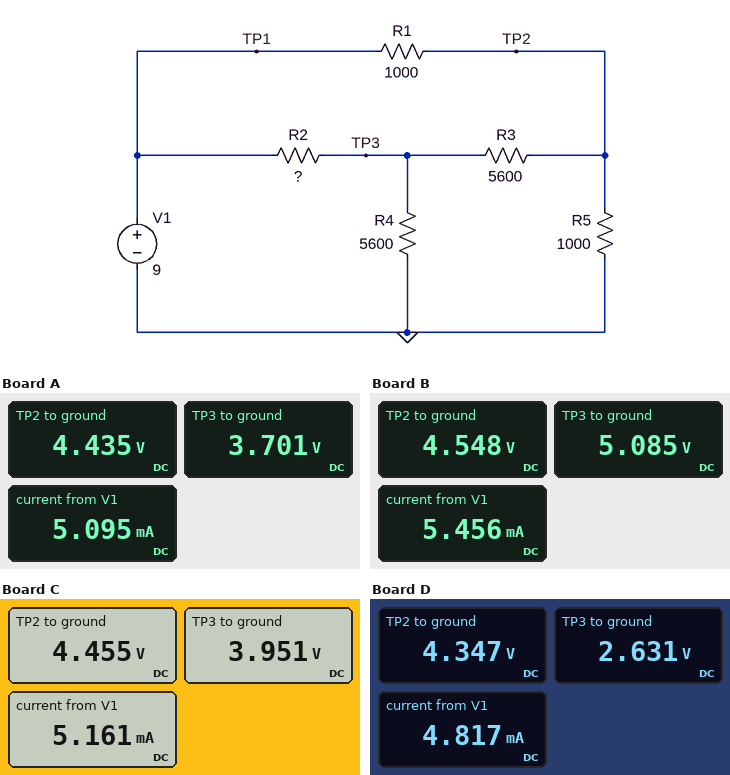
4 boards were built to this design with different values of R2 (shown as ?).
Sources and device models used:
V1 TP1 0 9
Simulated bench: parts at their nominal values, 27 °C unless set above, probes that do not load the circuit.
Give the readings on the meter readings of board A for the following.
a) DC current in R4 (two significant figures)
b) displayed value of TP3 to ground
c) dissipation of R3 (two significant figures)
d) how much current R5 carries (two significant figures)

660 µA
3.701 V
96 µW
4.4 mA
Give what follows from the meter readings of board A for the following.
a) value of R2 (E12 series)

10 kΩ
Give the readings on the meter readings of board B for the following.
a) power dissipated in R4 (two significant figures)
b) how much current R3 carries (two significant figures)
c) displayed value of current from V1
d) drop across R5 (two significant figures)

4.6 mW
96 µA
5.456 mA
4.5 V
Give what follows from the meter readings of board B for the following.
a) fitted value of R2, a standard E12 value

3.9 kΩ
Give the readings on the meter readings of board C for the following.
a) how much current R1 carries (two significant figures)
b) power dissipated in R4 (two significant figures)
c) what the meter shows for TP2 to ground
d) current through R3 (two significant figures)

4.5 mA
2.8 mW
4.455 V
90 µA
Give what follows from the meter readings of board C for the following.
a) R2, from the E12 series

8.2 kΩ
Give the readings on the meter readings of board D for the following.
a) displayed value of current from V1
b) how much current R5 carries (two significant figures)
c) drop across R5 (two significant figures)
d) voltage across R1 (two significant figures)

4.817 mA
4.3 mA
4.3 V
4.7 V
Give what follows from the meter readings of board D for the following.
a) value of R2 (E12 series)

39 kΩ
